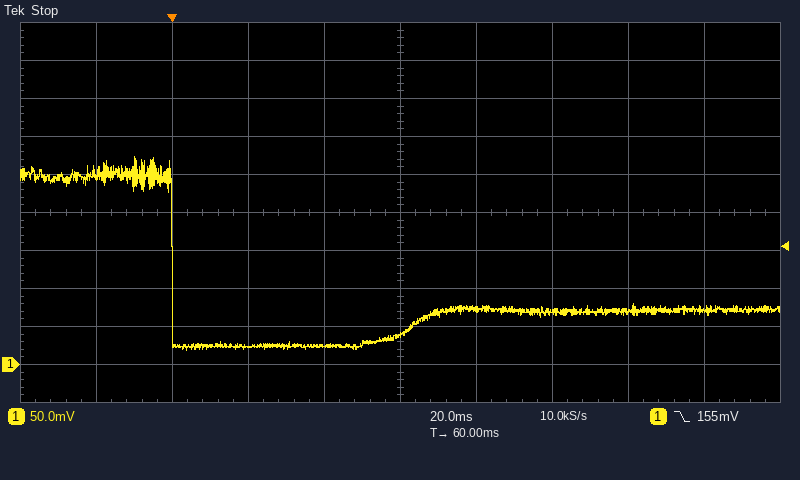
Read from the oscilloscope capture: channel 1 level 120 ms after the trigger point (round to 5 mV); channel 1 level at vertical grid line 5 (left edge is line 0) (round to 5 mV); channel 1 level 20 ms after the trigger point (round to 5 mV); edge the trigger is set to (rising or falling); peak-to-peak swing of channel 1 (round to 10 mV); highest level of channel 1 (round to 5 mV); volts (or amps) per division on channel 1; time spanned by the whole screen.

70 mV
40 mV
25 mV
falling
260 mV
275 mV
50 mV
200 ms
